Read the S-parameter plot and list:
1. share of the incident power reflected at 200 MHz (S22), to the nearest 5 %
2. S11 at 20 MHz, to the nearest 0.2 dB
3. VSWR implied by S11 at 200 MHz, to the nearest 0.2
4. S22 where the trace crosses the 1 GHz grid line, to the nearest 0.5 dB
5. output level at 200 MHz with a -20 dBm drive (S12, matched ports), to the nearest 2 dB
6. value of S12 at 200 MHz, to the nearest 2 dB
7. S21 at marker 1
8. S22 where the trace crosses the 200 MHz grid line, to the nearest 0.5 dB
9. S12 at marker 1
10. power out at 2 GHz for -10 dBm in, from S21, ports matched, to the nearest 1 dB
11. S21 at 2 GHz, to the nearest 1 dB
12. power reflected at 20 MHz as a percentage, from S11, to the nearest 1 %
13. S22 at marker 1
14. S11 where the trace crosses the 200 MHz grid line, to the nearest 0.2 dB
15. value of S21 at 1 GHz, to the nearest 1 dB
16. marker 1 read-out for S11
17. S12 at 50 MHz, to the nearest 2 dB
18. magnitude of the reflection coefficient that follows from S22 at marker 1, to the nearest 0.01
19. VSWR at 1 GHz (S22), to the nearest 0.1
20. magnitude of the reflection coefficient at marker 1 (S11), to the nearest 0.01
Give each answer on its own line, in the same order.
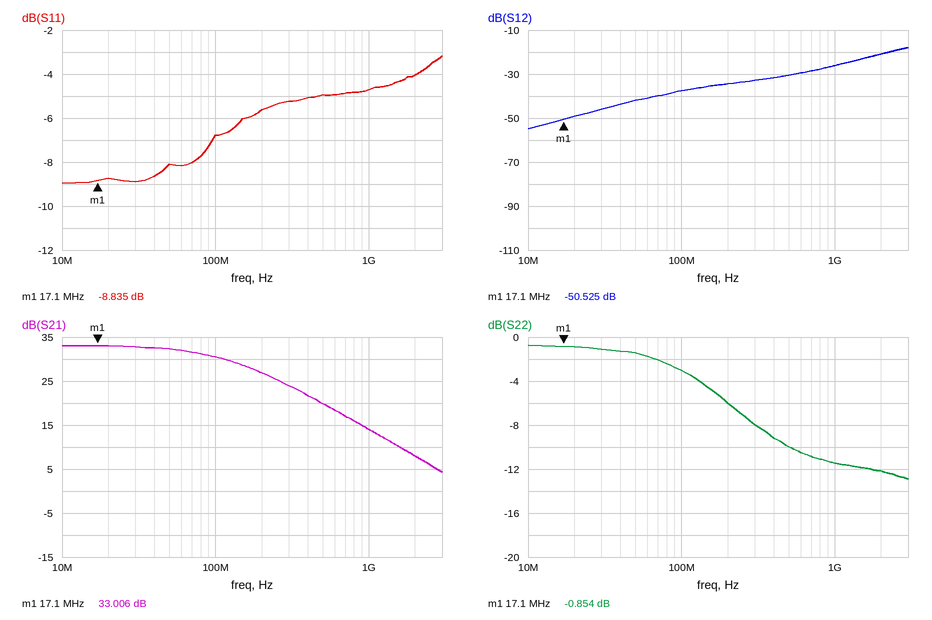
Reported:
25 %
-8.8 dB
3.2
-11.5 dB
-54 dBm
-34 dB
33.006 dB
-6.0 dB
-50.525 dB
-2 dBm
8 dB
13 %
-0.854 dB
-5.6 dB
14 dB
-8.835 dB
-42 dB
0.91
1.7
0.36
